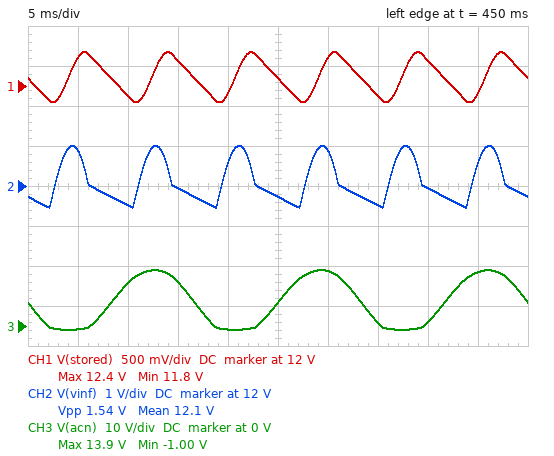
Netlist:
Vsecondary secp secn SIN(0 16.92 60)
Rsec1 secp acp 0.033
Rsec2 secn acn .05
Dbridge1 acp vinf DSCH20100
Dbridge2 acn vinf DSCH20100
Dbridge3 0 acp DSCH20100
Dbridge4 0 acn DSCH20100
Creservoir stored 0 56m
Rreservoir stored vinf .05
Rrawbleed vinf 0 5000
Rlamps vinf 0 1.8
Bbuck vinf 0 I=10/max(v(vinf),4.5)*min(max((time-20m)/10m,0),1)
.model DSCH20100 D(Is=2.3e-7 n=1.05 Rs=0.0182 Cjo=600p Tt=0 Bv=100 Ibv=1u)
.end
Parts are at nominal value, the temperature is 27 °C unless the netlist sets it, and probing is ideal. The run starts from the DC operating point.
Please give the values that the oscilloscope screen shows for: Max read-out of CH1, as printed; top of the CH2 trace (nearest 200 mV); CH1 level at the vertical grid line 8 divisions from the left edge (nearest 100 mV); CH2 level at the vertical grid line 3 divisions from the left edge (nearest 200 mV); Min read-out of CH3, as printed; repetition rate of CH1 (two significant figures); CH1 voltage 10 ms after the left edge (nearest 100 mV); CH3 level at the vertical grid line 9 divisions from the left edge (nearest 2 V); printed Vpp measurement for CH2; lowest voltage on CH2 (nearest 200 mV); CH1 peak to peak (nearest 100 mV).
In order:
12.4 V
13.0 V
12.3 V
12.0 V
-1.00 V
120 Hz
11.9 V
14 V
1.54 V
11.4 V
600 mV
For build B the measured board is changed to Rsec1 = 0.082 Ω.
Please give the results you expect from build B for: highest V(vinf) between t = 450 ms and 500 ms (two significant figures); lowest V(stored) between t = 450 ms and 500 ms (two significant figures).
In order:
12 V
11 V
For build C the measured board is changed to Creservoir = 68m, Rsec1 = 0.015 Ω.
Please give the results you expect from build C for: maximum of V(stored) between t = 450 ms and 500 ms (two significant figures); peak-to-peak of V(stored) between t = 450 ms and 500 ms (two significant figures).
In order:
13 V
540 mV
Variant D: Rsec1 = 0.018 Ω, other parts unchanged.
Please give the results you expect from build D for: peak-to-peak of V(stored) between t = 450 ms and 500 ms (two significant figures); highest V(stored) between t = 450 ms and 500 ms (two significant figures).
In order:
650 mV
13 V
